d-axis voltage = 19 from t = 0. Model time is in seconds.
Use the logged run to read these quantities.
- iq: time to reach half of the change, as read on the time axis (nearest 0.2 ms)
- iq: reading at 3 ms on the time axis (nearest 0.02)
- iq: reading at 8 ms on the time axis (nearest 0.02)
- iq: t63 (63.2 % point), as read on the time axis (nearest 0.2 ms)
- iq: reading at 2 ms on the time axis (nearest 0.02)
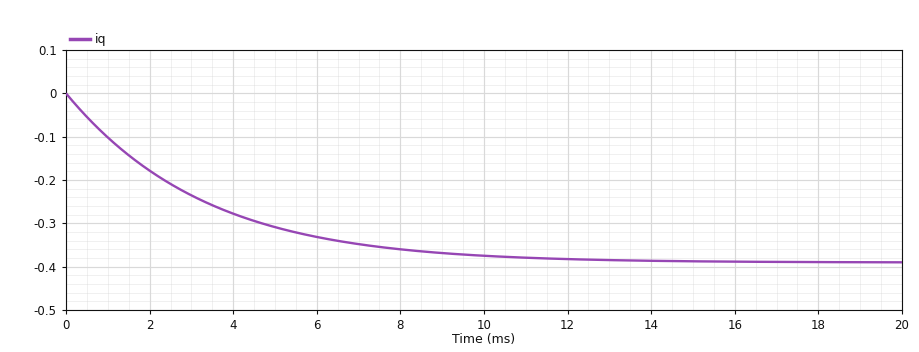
2.2 ms
-0.24
-0.36
3.2 ms
-0.18
